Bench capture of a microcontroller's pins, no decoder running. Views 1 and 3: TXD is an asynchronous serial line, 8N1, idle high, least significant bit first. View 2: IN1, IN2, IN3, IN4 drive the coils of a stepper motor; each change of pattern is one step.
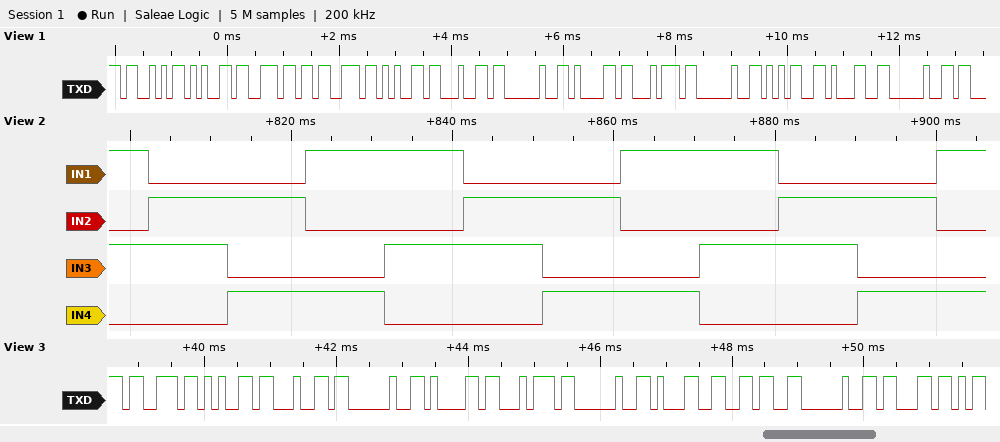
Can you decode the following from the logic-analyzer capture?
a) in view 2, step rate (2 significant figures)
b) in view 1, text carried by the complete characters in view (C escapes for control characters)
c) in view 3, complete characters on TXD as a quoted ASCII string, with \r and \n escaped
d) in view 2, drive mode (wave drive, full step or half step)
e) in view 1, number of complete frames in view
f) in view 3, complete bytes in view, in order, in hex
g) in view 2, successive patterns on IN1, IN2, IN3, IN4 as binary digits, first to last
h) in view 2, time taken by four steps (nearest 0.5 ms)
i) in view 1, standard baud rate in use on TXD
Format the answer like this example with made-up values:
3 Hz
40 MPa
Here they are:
100 steps/s
"Sensed at 51 "
"sed at 16 c"
full step
13
73 65 64 20 61 74 20 31 36 20 63
1010 0110 0101 1001 1010 0110 0101 1001 1010 0110 0101 1001
39.0 ms
9600 baud
